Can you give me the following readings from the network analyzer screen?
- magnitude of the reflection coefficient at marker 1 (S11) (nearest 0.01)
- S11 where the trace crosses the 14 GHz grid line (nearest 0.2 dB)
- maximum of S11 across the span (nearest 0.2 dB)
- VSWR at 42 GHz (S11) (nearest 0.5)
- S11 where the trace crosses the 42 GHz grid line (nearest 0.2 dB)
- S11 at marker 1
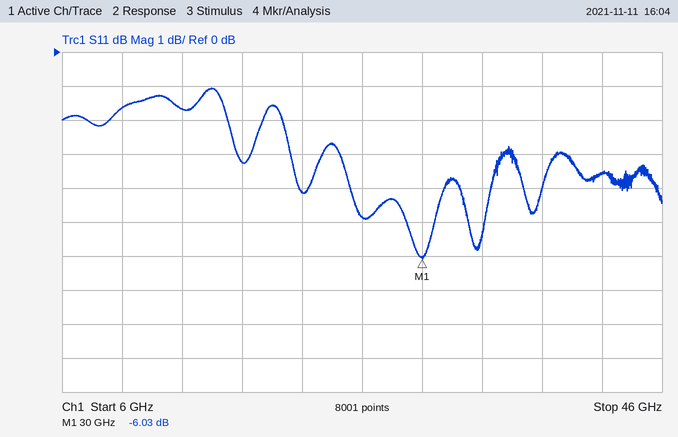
0.50
-1.6 dB
-1.0 dB
5.0
-3.6 dB
-6.03 dB
